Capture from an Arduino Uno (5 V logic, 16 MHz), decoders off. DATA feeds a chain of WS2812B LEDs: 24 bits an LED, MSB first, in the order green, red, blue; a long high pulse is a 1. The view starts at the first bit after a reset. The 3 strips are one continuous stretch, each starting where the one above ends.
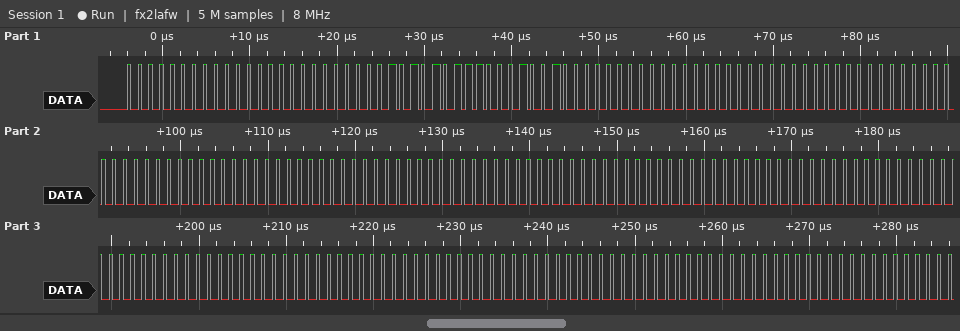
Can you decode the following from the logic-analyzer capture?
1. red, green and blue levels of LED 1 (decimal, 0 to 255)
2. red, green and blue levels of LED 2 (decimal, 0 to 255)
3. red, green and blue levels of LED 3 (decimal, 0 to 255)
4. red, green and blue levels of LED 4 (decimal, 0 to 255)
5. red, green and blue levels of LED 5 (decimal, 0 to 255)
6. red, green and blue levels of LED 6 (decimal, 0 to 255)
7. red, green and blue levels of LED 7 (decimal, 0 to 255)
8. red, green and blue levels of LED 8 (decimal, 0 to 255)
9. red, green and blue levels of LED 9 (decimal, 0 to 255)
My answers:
0, 0, 0
137, 171, 0
0, 0, 0
0, 0, 0
0, 0, 0
0, 0, 0
0, 0, 0
0, 0, 0
0, 0, 0
